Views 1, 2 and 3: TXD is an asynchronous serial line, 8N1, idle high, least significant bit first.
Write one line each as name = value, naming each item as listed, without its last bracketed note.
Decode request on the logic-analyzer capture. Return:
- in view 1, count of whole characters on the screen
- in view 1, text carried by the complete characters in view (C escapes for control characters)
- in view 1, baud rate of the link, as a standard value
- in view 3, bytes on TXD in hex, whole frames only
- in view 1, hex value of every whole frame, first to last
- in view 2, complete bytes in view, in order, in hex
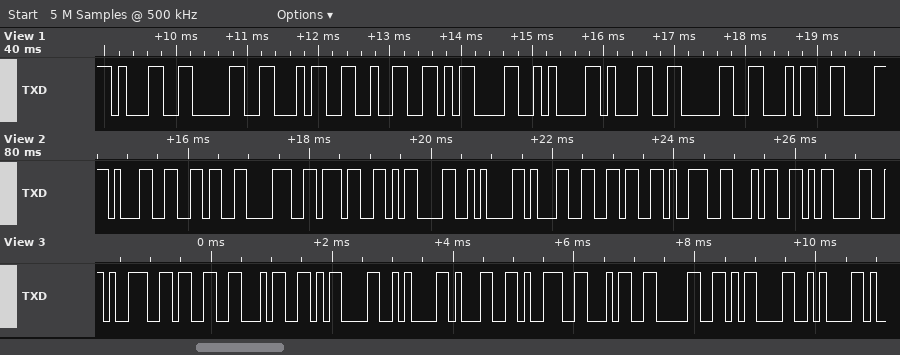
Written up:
in view 1, count of whole characters on the screen = 9
in view 1, text carried by the complete characters in view = "1042\r\n104"
in view 1, baud rate of the link, as a standard value = 9600 baud
in view 3, bytes on TXD in hex, whole frames only = 39 33 34 0D 0A 31 39 34 30 0D 0A
in view 1, hex value of every whole frame, first to last = 31 30 34 32 0D 0A 31 30 34
in view 2, complete bytes in view, in order, in hex = 0x31 0x36 0x38 0x37 0x0D 0x0A 0x31 0x36 0x39 0x34 0x0D
